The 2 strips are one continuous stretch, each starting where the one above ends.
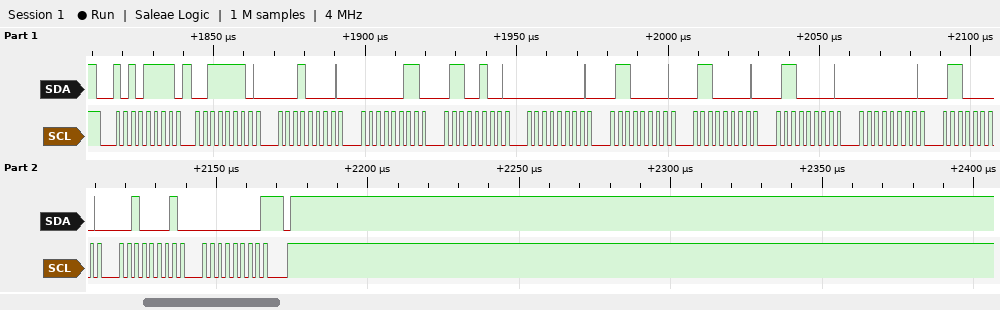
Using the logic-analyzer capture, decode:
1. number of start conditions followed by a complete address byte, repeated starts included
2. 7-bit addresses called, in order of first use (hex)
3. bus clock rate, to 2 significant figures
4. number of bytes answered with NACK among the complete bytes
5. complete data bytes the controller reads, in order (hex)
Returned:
1
0x57
400 kHz
1
3E 10 03 64 00 60 60 60 00 60 21 00
